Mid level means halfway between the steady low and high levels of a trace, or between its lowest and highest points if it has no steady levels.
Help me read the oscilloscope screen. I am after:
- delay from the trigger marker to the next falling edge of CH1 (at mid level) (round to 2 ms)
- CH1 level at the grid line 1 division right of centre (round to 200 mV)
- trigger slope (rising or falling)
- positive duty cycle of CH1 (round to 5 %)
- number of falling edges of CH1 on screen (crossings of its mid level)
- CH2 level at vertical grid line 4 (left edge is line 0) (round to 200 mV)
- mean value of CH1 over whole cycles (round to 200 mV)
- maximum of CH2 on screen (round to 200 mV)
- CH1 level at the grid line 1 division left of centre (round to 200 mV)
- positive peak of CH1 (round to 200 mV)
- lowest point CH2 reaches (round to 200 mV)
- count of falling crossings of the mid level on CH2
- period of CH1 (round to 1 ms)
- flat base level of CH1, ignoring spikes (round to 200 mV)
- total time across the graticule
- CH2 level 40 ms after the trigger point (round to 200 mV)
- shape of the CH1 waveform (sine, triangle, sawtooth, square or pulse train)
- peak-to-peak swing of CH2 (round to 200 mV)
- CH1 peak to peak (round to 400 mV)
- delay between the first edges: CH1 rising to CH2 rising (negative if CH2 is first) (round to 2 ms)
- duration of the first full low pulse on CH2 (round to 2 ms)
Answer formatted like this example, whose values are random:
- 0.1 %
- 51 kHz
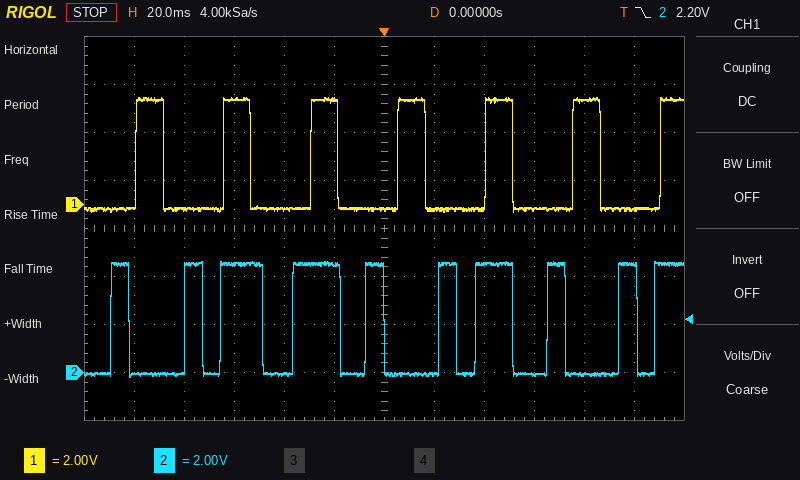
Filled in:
- 16 ms
- -200 mV
- falling
- 30 %
- 6
- 0.0 V
- 1.2 V
- 4.6 V
- 4.4 V
- 4.4 V
- -200 mV
- 9
- 35 ms
- -200 mV
- 240 ms
- 4.6 V
- pulse train
- 4.8 V
- 4.8 V
- -10 ms
- 22 ms
